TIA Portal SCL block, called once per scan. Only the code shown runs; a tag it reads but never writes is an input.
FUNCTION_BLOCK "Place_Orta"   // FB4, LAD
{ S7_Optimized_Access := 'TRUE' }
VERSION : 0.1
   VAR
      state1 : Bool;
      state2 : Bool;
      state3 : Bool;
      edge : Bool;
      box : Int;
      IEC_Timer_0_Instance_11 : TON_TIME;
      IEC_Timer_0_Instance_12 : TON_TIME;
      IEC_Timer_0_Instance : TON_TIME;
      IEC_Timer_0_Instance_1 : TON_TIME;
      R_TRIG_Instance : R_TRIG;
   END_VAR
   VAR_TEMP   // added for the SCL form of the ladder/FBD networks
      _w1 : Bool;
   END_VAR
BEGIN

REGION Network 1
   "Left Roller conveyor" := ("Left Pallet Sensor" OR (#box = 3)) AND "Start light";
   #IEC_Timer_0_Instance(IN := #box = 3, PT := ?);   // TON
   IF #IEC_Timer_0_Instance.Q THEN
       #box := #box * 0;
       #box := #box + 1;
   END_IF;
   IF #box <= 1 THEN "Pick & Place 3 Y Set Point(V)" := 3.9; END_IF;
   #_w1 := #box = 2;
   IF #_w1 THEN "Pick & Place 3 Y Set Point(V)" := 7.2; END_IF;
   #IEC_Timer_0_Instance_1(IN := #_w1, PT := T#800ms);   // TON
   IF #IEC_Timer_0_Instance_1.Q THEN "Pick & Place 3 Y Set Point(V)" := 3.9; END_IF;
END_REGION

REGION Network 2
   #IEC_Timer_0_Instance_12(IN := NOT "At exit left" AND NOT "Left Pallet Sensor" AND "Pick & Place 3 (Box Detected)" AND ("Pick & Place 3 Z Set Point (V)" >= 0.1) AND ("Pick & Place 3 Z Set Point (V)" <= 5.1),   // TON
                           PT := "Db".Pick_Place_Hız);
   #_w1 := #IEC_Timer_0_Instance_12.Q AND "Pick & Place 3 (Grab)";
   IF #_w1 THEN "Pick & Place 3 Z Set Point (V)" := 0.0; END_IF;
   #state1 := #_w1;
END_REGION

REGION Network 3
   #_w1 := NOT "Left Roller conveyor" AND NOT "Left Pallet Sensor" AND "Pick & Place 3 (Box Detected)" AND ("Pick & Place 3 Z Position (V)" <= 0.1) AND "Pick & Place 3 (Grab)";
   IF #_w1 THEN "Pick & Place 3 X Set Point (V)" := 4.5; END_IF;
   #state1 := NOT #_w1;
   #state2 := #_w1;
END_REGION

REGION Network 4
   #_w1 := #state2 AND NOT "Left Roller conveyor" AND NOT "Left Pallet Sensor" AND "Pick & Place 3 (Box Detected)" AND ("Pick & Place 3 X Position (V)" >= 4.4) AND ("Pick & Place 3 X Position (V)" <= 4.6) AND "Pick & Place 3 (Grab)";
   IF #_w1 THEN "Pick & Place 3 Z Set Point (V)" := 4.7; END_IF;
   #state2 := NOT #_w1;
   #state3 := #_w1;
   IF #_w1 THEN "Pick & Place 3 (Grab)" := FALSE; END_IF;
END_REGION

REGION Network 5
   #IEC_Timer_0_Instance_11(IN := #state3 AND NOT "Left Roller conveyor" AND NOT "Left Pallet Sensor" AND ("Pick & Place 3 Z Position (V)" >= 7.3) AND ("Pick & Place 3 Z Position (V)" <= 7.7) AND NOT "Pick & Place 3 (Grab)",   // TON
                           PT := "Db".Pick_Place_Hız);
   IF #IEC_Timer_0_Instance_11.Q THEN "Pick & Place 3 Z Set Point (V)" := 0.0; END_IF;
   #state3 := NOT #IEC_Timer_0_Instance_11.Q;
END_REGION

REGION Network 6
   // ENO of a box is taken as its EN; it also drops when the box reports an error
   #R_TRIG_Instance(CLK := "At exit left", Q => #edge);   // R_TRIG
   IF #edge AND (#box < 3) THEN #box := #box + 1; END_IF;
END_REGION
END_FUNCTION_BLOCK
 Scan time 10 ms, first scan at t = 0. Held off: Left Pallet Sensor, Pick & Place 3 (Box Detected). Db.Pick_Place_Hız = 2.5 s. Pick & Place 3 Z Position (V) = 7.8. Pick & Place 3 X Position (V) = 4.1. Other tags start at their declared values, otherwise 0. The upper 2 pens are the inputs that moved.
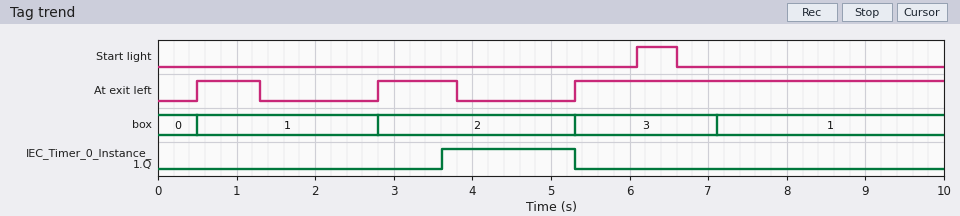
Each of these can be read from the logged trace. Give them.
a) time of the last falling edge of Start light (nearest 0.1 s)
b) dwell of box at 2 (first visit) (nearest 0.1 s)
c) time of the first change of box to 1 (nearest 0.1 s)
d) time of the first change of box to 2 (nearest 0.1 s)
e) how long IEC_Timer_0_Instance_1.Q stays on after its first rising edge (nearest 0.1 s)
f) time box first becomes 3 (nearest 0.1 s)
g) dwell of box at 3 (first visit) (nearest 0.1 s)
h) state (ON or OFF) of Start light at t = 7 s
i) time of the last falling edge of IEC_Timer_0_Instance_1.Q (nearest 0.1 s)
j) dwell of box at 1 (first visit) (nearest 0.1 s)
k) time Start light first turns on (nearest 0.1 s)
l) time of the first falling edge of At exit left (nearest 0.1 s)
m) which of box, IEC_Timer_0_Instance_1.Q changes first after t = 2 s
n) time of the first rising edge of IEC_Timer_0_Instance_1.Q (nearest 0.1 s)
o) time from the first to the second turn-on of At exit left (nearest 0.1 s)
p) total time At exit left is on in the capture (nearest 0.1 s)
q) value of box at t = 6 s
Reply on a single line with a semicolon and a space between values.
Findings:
6.6 s; 2.5 s; 0.5 s; 2.8 s; 1.7 s; 5.3 s; 1.8 s; OFF; 5.3 s; 2.3 s; 6.1 s; 1.3 s; box; 3.6 s; 2.3 s; 6.5 s; 3
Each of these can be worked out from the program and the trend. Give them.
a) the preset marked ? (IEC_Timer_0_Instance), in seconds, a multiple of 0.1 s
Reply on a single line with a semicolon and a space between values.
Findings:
1.8 s
